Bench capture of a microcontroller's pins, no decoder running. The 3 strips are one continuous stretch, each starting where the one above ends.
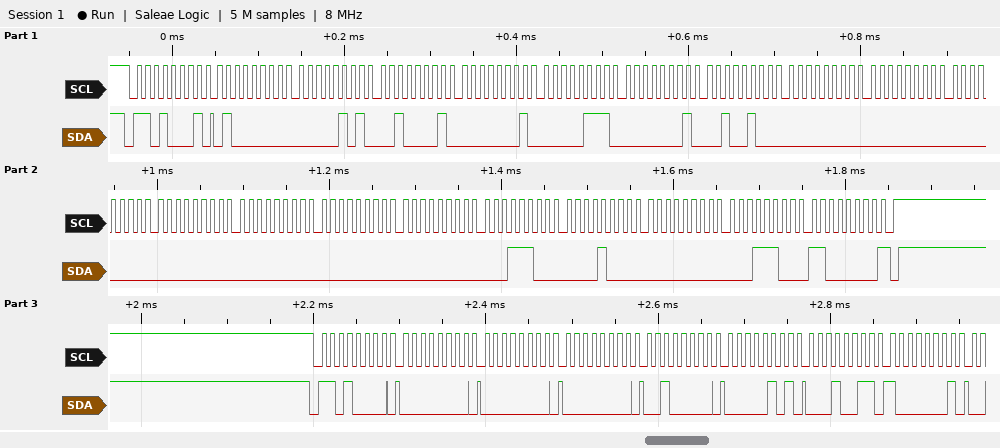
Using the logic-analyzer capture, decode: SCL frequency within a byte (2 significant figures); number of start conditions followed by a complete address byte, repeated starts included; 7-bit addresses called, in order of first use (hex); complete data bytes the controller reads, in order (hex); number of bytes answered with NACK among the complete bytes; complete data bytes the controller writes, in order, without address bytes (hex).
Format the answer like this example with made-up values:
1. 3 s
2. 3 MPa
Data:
1. 100 kHz
2. 2
3. 0x68
4. 40 05 21 01 07 01 24 00 00 00 00 00 00 00 1C 08 00 1C C0
5. 1
6. 00 00 00 20 05 13 81
